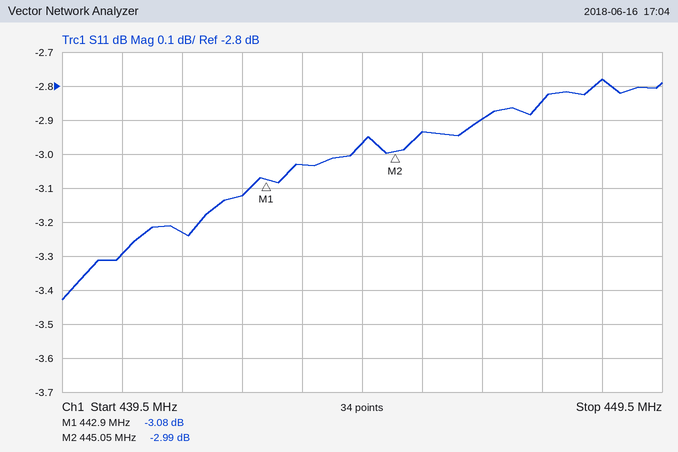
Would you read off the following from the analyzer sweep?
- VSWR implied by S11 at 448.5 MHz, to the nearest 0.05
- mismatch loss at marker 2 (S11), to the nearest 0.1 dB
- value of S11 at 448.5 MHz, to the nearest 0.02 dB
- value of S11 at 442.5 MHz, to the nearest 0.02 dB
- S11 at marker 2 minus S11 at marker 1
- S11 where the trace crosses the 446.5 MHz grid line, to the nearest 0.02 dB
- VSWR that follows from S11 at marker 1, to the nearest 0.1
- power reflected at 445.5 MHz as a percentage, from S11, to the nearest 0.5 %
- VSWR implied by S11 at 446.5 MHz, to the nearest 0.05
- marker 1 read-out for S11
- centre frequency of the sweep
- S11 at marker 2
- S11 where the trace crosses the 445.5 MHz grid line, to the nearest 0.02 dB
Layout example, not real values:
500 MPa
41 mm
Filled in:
6.30
3.0 dB
-2.78 dB
-3.12 dB
0.09 dB
-2.90 dB
5.7
51.0 %
6.05
-3.08 dB
444.5 MHz
-2.99 dB
-2.94 dB
